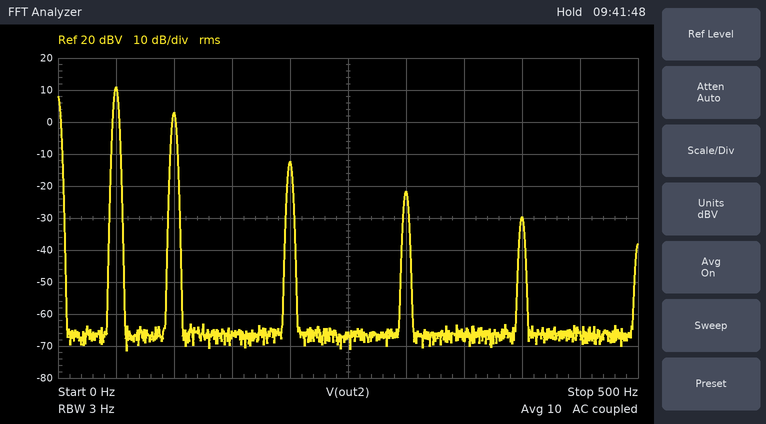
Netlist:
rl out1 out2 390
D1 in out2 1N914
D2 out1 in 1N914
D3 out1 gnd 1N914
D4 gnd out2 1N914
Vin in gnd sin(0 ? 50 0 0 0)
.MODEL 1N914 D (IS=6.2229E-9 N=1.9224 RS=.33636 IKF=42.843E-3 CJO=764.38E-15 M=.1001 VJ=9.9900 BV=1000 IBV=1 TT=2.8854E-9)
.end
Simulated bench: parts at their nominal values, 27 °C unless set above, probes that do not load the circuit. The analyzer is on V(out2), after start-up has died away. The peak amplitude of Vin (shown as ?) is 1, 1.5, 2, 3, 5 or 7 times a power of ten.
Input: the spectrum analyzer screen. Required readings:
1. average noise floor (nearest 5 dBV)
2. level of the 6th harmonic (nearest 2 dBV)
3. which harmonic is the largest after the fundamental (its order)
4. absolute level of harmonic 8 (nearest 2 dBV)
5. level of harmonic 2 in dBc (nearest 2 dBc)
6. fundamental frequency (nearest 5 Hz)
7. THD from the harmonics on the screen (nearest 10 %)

-65 dBV
-22 dBV
2
-30 dBV
-8 dBc
50 Hz
40 %
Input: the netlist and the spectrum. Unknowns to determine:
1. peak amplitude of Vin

10 V
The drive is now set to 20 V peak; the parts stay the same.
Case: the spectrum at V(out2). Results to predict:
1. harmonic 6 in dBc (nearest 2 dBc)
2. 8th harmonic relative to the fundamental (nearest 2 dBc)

-30 dBc
-36 dBc
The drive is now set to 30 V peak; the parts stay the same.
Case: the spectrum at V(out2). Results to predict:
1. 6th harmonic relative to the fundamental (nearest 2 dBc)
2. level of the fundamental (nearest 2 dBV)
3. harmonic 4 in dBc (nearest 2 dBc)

-30 dBc
20 dBV
-22 dBc
